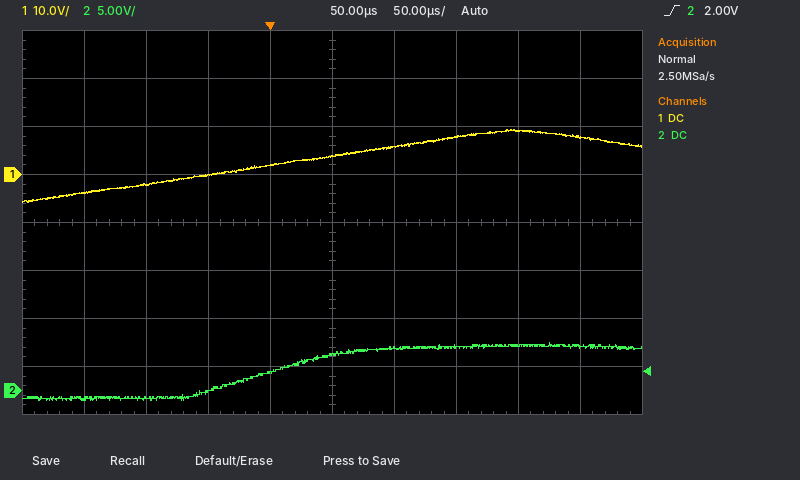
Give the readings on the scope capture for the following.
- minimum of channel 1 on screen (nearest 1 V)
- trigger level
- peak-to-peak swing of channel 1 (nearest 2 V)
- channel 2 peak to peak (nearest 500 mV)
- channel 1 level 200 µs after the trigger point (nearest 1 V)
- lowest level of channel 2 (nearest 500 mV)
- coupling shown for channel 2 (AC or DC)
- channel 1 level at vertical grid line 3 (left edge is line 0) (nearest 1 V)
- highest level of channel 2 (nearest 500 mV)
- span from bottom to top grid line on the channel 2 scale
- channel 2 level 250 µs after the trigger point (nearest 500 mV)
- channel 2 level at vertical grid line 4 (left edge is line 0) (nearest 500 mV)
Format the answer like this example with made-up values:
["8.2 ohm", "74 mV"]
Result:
["-6 V", "2.00 V", "16 V", "6.0 V", "9 V", "-1.0 V", "DC", "0 V", "5.0 V", "40 V", "4.5 V", "2.0 V"]
